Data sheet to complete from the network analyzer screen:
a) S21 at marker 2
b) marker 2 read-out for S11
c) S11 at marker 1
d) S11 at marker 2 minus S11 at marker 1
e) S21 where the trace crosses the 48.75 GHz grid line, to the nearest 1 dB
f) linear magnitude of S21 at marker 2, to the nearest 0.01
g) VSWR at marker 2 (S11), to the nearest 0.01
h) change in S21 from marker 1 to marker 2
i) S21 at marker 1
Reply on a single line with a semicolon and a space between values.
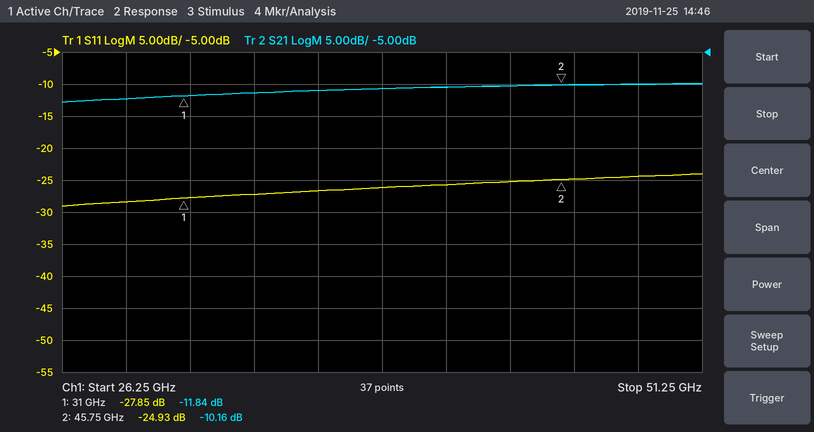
-10.16 dB; -24.93 dB; -27.85 dB; 2.92 dB; -10 dB; 0.31; 1.12; 1.68 dB; -11.84 dB
